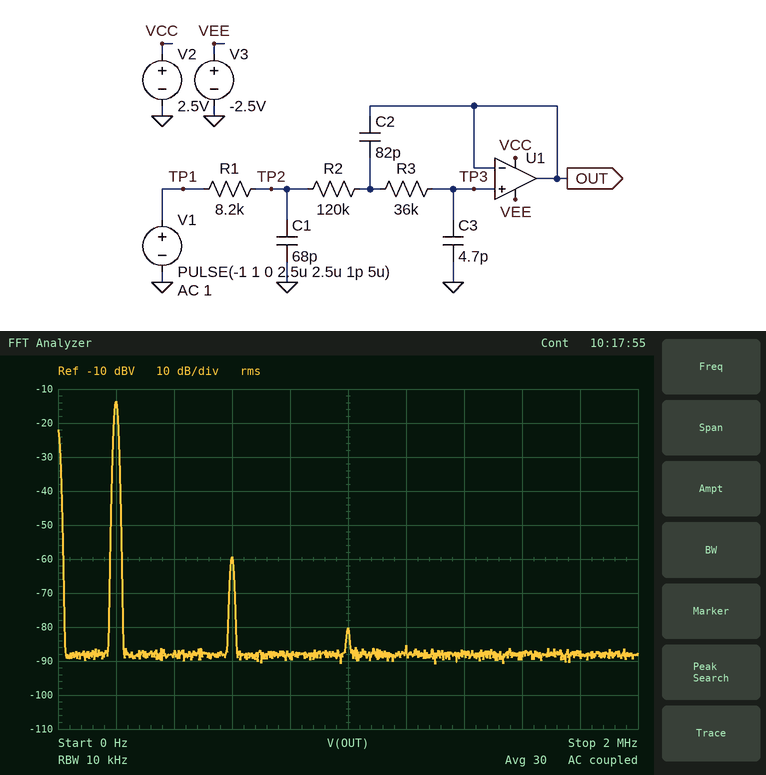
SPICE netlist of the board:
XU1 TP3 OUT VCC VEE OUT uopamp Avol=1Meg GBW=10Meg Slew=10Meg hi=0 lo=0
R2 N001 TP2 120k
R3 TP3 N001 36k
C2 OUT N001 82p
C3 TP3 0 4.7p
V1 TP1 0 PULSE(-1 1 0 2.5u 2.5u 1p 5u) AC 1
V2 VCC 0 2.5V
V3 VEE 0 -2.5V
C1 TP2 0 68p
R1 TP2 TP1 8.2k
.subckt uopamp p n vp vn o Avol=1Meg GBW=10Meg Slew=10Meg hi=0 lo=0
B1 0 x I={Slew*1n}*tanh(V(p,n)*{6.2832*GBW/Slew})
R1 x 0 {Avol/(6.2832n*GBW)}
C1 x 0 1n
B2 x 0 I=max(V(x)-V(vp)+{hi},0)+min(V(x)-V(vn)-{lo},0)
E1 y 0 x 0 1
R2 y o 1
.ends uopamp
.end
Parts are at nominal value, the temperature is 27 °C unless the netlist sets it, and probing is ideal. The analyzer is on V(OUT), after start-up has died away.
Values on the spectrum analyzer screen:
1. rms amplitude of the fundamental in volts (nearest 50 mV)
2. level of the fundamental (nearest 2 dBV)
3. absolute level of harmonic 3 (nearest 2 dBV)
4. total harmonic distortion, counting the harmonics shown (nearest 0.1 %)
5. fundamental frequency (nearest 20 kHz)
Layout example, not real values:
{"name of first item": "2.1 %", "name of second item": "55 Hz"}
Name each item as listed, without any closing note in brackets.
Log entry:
{"rms amplitude of the fundamental in volts": "200 mV", "level of the fundamental": "-14 dBV", "absolute level of harmonic 3": "-60 dBV", "total harmonic distortion, counting the harmonics shown": "0.5 %", "fundamental frequency": "200 kHz"}
